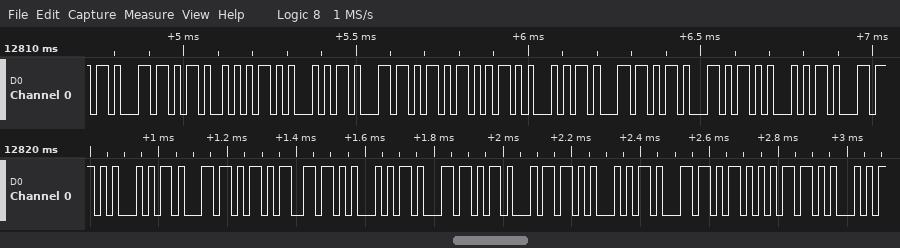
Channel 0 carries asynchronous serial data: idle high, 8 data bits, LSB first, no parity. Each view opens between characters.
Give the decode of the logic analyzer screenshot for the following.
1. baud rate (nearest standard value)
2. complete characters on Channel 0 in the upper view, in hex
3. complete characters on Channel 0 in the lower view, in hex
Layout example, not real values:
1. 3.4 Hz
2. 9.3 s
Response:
1. 57600 baud
2. 8B, 6B, AA, 45, 8B, 6B, AB, 45, 8B, 6B, AC, 45, 8B
3. 45, 8B, 6B, B3, 45, 8B, 6B, B4, 45, 8B, 6B, B5, 45
